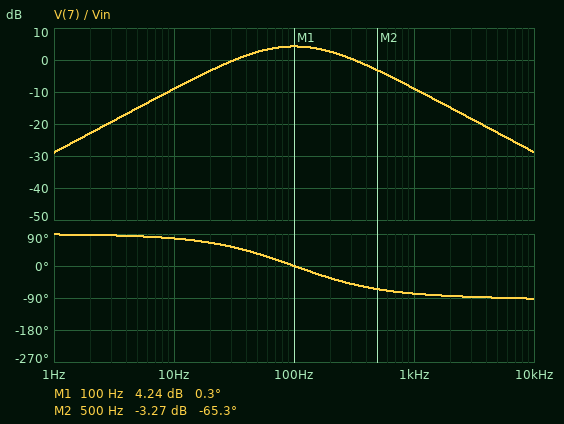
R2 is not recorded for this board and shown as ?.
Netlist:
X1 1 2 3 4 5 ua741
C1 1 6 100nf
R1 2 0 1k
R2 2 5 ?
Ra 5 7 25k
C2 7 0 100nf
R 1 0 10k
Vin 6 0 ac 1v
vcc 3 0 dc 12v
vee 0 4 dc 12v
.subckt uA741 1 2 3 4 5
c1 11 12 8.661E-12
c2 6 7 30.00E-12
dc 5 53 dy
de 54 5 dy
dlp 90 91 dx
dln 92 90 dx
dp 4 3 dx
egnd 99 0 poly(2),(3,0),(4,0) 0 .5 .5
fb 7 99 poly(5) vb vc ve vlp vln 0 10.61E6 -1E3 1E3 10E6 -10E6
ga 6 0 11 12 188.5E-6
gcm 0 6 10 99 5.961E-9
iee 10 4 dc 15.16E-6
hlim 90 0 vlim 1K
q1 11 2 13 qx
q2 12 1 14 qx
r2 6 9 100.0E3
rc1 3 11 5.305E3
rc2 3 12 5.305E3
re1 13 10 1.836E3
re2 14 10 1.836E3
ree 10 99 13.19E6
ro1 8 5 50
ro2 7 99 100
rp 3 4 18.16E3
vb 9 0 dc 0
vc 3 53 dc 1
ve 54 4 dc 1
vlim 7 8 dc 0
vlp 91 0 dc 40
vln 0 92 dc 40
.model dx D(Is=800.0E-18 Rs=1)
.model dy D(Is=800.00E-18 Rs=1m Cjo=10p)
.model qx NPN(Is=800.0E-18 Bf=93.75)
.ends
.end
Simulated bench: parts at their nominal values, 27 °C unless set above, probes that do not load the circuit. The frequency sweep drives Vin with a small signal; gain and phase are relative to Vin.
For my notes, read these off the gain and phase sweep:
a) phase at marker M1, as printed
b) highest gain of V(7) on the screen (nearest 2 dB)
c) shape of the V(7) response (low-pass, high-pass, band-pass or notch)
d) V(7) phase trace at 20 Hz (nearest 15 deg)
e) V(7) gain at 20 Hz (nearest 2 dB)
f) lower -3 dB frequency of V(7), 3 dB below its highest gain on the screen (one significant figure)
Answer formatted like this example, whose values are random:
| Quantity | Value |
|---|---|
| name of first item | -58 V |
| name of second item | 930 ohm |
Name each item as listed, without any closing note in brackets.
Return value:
| Quantity | Value |
|---|---|
| phase at marker M1, as printed | 0.3 deg |
| highest gain of V(7) on the screen | 4 dB |
| shape of the V(7) response | band-pass |
| V(7) phase trace at 20 Hz | 60 deg |
| V(7) gain at 20 Hz | -4 dB |
| lower -3 dB frequency of V(7), 3 dB below its highest gain on the screen | 40 Hz |
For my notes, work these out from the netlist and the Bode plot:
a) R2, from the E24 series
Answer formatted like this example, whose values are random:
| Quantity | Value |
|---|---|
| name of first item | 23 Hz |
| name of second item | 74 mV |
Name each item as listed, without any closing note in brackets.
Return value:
| Quantity | Value |
|---|---|
| R2, from the E24 series | 4.7 kΩ |
